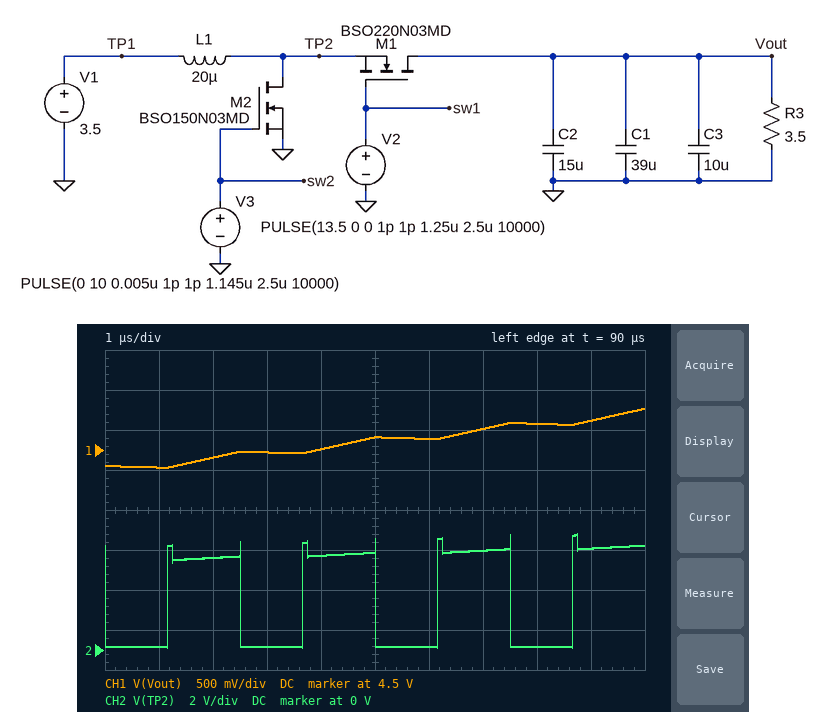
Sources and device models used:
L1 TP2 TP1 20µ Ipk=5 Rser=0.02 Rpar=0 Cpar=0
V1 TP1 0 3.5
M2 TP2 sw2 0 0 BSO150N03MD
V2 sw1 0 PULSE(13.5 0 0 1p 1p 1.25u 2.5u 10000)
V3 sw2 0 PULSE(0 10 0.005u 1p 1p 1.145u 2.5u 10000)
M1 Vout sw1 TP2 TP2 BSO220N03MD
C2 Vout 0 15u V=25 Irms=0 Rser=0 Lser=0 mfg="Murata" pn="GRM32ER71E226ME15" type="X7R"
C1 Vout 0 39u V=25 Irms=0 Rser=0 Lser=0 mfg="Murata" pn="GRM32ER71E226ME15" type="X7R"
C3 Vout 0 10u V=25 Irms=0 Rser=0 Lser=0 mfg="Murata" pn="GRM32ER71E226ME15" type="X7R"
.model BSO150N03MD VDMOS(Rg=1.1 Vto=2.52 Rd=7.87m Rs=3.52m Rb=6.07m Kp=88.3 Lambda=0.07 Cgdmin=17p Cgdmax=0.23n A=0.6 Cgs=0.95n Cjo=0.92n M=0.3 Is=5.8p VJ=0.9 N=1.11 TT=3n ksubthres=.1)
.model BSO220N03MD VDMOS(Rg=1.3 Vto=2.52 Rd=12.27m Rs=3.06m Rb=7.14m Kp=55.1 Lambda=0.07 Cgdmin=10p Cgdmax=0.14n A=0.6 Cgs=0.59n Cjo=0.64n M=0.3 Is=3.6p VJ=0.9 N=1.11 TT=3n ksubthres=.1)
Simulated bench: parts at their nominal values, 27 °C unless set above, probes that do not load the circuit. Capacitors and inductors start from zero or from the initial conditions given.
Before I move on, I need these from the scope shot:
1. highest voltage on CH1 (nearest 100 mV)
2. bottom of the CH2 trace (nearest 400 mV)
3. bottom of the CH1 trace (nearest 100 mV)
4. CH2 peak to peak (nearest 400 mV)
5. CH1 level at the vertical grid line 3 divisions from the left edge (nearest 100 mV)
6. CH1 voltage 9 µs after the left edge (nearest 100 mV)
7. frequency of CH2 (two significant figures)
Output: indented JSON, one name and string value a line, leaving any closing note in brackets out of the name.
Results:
{
  "highest voltage on CH1": "5.0 V",
  "bottom of the CH2 trace": "0 V",
  "bottom of the CH1 trace": "4.3 V",
  "CH2 peak to peak": "5.6 V",
  "CH1 level at the vertical grid line 3 divisions from the left edge": "4.5 V",
  "CH1 voltage 9 µs after the left edge": "4.9 V",
  "frequency of CH2": "400 kHz"
}
